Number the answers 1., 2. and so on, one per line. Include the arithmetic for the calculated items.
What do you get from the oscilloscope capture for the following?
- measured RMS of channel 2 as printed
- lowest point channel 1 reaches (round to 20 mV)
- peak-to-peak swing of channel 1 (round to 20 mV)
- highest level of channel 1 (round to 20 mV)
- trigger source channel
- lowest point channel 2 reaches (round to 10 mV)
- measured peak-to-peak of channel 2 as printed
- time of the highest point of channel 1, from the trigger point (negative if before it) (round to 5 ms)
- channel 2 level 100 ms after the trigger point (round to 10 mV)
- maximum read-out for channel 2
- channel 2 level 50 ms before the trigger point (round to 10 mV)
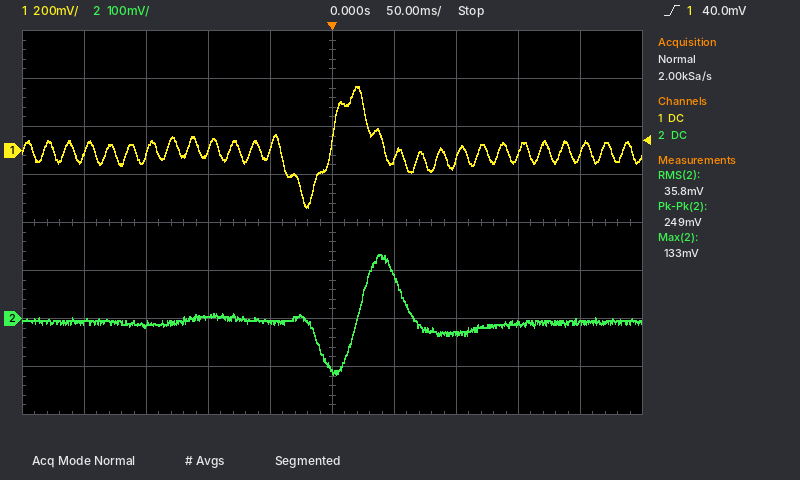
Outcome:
1. 35.8 mV
2. -240 mV
3. 260 mV − (-240 mV) = 500 mV
4. 260 mV
5. channel 1
6. -120 mV
7. 249 mV
8. +20 ms
9. -30 mV
10. 133 mV
11. -10 mV
